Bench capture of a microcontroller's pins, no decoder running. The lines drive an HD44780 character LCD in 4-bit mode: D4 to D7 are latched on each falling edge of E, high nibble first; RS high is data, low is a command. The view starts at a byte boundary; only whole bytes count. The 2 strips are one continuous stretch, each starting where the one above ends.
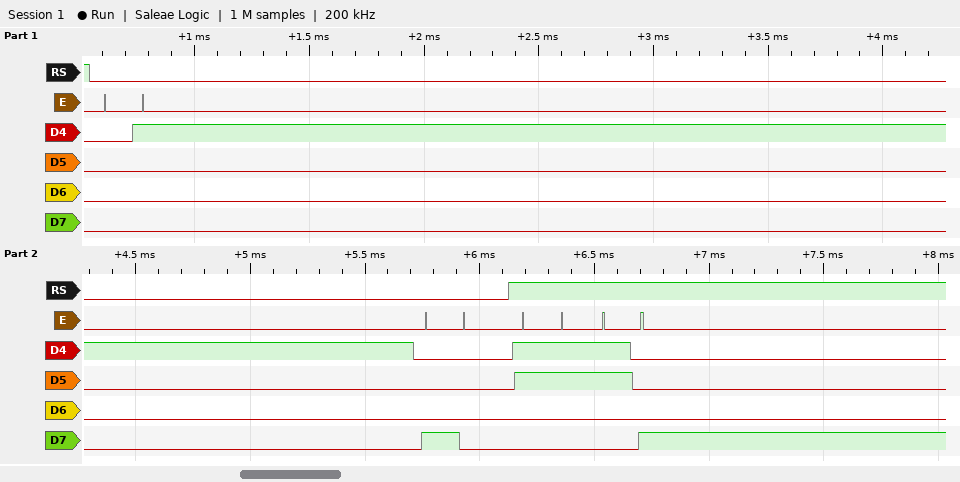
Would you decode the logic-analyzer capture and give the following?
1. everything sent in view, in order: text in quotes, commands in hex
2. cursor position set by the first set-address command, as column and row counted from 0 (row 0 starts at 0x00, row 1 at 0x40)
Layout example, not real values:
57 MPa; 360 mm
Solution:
0x01 0x80 "38"; column 0, row 0
